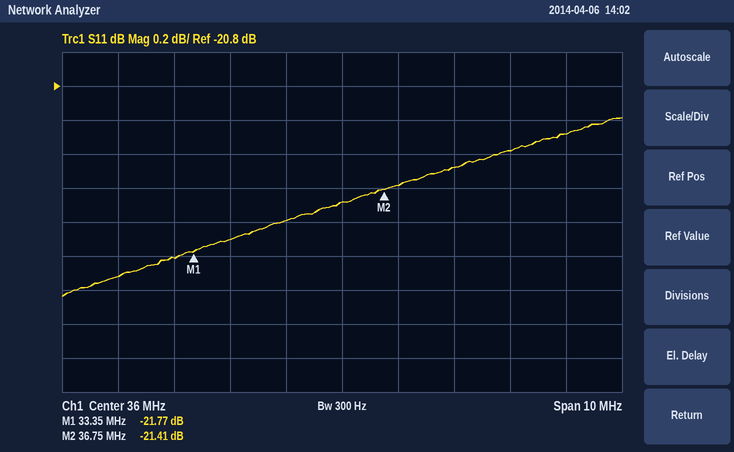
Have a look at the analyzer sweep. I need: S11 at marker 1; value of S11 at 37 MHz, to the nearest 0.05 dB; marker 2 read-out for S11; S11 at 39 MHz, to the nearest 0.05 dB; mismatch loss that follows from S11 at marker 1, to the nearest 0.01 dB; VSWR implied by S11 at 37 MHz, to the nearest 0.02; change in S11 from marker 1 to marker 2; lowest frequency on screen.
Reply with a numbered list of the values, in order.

1. -21.77 dB
2. -21.40 dB
3. -21.41 dB
4. -21.20 dB
5. 0.03 dB
6. 1.18
7. 0.36 dB
8. 31 MHz
